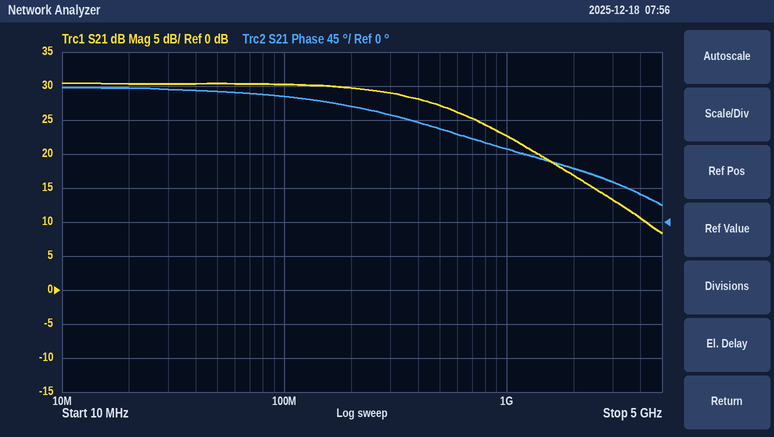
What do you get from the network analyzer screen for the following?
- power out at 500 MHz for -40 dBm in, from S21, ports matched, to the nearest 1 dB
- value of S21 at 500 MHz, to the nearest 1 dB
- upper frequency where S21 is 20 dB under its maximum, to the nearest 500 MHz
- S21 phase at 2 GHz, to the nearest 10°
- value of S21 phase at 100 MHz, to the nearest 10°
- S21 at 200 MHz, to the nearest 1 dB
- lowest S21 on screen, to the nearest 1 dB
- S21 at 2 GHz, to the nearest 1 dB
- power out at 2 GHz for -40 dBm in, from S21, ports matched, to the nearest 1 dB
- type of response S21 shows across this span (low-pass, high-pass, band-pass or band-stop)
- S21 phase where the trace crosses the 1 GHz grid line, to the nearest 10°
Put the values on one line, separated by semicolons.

-13 dBm; 27 dB; 4.0 GHz; 70°; 170°; 30 dB; 8 dB; 17 dB; -23 dBm; low-pass; 100°
